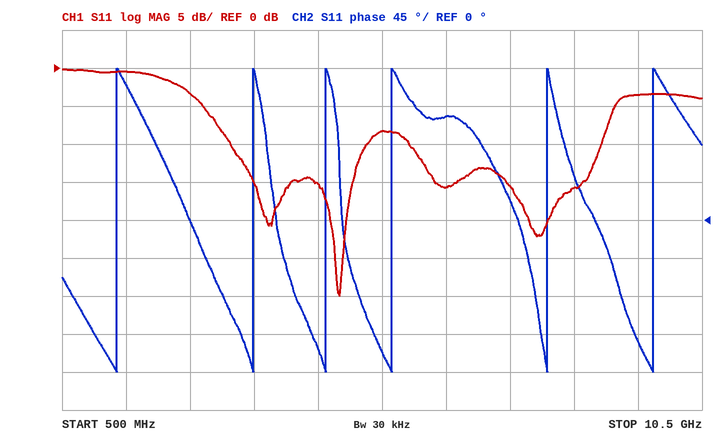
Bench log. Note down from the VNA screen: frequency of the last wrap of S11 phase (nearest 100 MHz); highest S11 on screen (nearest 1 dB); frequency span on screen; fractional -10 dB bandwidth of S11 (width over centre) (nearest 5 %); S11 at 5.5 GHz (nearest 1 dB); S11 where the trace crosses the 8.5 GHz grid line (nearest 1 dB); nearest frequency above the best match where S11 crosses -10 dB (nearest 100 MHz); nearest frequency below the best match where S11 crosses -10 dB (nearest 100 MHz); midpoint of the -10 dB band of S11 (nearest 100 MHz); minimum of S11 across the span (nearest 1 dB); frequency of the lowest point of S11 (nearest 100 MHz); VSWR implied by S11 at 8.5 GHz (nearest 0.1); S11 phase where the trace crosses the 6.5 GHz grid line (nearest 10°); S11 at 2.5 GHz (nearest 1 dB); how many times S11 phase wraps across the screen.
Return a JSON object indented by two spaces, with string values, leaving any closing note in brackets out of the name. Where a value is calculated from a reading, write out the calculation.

{
  "frequency of the last wrap of S11 phase": "9.7 GHz",
  "highest S11 on screen": "0 dB",
  "frequency span on screen": "10 GHz",
  "fractional -10 dB bandwidth of S11 (width over centre)": "2.2 GHz / 4.2 GHz ≈ 52.4 %, so 50 % to the nearest 5 %",
  "S11 at 5.5 GHz": "-8 dB",
  "S11 where the trace crosses the 8.5 GHz grid line": "-16 dB",
  "nearest frequency above the best match where S11 crosses -10 dB": "5.3 GHz",
  "nearest frequency below the best match where S11 crosses -10 dB": "3.1 GHz",
  "midpoint of the -10 dB band of S11": "4.2 GHz",
  "minimum of S11 across the span": "-30 dB",
  "frequency of the lowest point of S11": "4.8 GHz",
  "VSWR implied by S11 at 8.5 GHz": "|Γ| = 10^(-16/20) = 0.1585; VSWR = (1 + 0.1585)/(1 − 0.1585) ≈ 1.4",
  "S11 phase where the trace crosses the 6.5 GHz grid line": "120°",
  "S11 at 2.5 GHz": "-3 dB",
  "how many times S11 phase wraps across the screen": "6"
}
